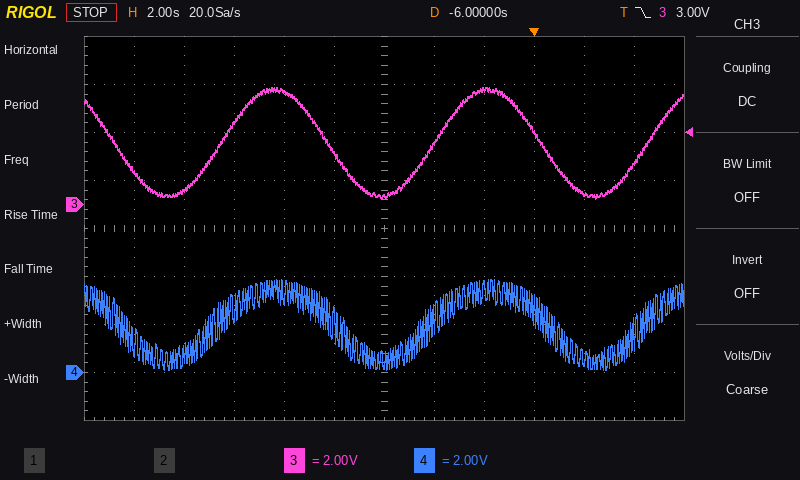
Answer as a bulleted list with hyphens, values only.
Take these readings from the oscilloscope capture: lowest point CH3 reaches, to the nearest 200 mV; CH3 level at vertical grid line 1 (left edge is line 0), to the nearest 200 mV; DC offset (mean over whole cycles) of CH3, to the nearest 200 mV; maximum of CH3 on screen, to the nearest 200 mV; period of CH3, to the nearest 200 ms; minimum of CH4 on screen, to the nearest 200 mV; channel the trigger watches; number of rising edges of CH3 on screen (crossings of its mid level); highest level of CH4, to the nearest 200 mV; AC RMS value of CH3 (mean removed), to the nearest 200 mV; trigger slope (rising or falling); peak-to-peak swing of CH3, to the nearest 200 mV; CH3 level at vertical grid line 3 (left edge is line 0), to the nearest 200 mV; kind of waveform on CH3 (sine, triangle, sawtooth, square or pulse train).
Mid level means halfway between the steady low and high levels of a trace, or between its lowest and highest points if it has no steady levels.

- 200 mV
- 1.4 V
- 2.6 V
- 4.8 V
- 8.6 s
- 200 mV
- CH3
- 3
- 3.8 V
- 1.6 V
- falling
- 4.6 V
- 3.4 V
- sine
